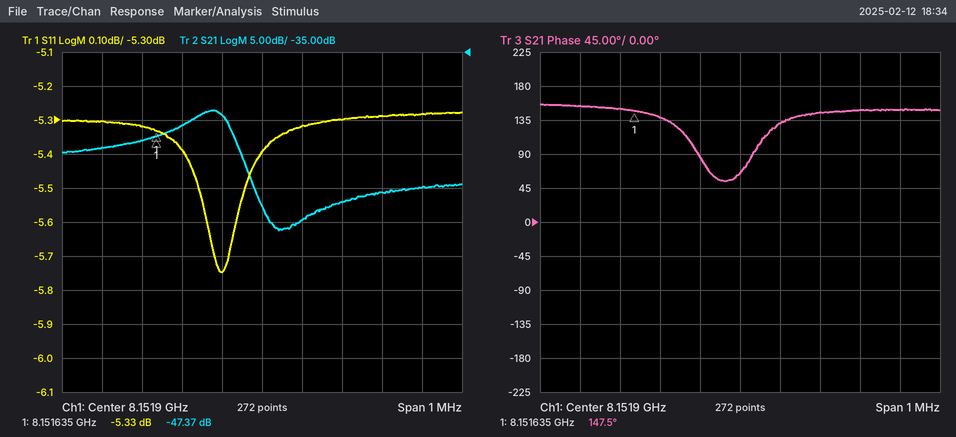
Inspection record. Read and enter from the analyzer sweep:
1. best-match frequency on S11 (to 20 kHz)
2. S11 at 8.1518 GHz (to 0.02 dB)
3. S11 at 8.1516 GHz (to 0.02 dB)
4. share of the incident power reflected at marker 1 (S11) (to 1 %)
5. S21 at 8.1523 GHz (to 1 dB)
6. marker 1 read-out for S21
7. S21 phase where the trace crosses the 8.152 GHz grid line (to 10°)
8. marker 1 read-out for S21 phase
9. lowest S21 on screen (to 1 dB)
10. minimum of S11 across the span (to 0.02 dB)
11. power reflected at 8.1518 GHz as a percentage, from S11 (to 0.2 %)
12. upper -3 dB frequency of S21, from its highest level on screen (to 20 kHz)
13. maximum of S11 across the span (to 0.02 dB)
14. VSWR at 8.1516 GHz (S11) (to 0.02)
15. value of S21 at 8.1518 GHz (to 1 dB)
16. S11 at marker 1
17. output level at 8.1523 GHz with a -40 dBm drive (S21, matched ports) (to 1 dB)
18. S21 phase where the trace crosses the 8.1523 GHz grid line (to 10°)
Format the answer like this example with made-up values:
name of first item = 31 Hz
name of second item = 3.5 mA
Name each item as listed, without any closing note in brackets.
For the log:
best-match frequency on S11 = 8.15180 GHz
S11 at 8.1518 GHz = -5.74 dB
S11 at 8.1516 GHz = -5.32 dB
share of the incident power reflected at marker 1 (S11) = 29 %
S21 at 8.1523 GHz = -55 dB
marker 1 read-out for S21 = -47.37 dB
S21 phase where the trace crosses the 8.152 GHz grid line = 130°
marker 1 read-out for S21 phase = 147.5°
lowest S21 on screen = -61 dB
minimum of S11 across the span = -5.74 dB
power reflected at 8.1518 GHz as a percentage, from S11 = 26.6 %
upper -3 dB frequency of S21, from its highest level on screen = 8.15182 GHz
maximum of S11 across the span = -5.28 dB
VSWR at 8.1516 GHz (S11) = 3.36
value of S21 at 8.1518 GHz = -44 dB
S11 at marker 1 = -5.33 dB
output level at 8.1523 GHz with a -40 dBm drive (S21, matched ports) = -95 dBm
S21 phase where the trace crosses the 8.1523 GHz grid line = 150°
